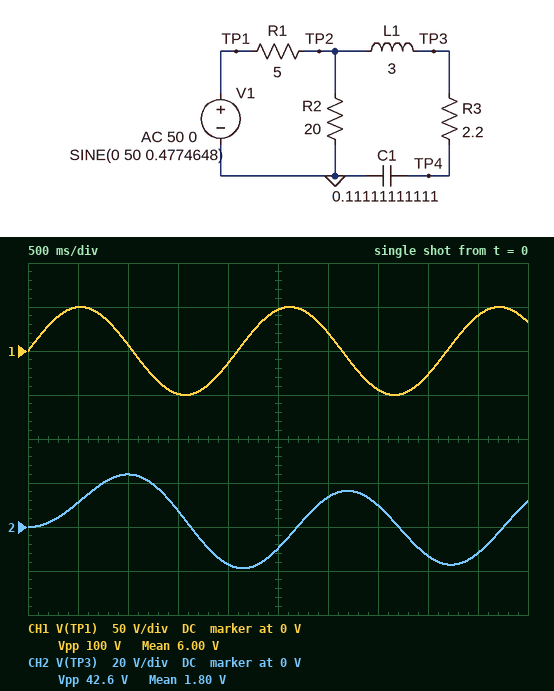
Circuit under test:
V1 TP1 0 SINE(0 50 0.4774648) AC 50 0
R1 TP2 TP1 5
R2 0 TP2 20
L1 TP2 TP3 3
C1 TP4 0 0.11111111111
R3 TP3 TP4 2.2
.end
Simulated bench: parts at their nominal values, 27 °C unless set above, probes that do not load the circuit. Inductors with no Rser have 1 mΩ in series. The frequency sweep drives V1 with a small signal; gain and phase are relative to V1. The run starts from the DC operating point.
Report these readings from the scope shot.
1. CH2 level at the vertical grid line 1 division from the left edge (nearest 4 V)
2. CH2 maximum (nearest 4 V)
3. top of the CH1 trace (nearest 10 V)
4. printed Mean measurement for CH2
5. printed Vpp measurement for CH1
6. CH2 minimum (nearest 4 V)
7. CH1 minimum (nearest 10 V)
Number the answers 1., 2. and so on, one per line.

1. 12 V
2. 24 V
3. 50 V
4. 1.80 V
5. 100 V
6. -20 V
7. -50 V
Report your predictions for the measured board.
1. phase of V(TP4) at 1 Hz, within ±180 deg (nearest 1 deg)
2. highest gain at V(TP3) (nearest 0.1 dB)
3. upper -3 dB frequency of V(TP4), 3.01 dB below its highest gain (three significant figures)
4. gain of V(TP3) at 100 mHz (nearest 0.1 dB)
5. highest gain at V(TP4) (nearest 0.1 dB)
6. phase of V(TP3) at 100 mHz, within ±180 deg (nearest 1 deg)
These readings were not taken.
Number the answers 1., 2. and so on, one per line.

1. -160 deg
2. -1.3 dB
3. 308 mHz
4. -1.6 dB
5. -1.6 dB
6. -18 deg
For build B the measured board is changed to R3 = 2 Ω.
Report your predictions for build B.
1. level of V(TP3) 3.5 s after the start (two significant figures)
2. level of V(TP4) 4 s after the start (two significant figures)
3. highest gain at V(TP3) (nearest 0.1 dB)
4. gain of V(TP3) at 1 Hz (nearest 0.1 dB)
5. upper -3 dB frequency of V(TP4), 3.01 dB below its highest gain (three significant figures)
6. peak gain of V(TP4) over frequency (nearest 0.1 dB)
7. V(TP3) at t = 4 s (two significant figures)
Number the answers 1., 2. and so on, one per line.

1. 10 V
2. -3.2 V
3. -1.2 dB
4. -19.4 dB
5. 311 mHz
6. -1.4 dB
7. -12 V
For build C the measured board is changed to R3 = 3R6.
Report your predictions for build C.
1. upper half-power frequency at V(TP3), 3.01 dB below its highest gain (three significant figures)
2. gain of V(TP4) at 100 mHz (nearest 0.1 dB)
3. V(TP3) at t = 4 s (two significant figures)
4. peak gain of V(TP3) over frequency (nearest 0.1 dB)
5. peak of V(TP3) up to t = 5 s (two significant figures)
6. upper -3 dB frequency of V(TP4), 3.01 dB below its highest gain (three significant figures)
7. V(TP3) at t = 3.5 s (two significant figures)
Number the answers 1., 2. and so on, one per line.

1. 332 mHz
2. -2.1 dB
3. -18 V
4. -1.8 dB
5. 25 V
6. 266 mHz
7. 5.3 V
